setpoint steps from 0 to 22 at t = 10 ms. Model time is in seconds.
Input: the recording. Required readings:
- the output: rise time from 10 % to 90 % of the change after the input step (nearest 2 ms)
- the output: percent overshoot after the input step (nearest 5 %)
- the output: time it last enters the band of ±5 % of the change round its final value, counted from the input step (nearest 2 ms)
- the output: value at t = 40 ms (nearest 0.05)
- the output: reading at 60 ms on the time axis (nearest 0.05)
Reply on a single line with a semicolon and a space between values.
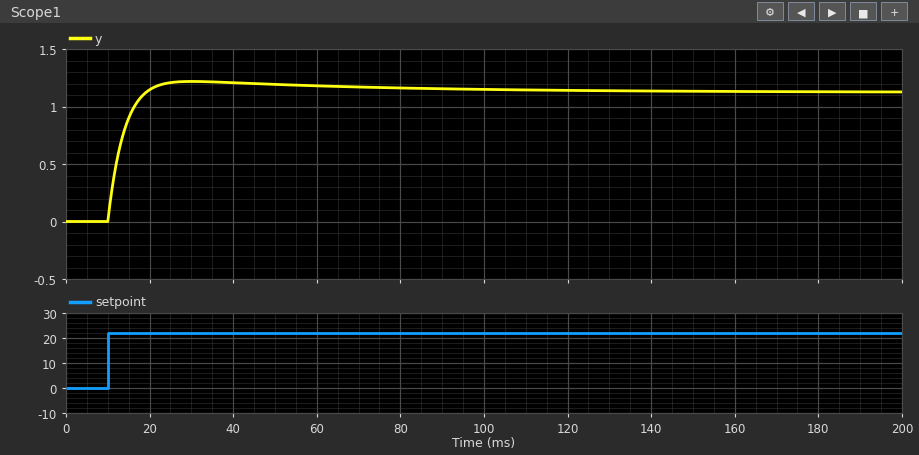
6 ms; 10 %; 50 ms; 1.20; 1.20
